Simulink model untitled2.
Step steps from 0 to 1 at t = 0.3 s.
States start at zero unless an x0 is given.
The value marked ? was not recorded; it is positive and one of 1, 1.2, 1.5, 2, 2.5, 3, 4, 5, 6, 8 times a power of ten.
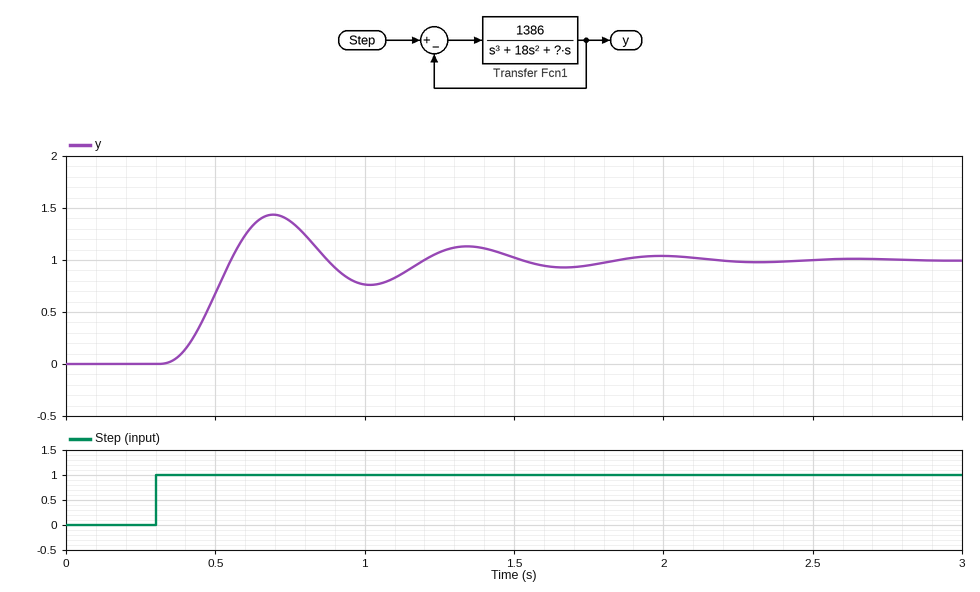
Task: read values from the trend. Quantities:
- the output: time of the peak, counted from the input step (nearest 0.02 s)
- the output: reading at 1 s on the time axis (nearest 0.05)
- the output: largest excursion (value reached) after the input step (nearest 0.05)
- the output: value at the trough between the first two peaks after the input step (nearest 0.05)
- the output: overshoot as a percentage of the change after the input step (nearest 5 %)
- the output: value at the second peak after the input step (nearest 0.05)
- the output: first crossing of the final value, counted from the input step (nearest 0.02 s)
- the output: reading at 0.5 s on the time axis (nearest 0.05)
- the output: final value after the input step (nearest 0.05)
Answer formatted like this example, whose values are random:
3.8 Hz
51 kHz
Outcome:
0.40 s
0.75
1.45
0.75
45 %
1.15
0.26 s
0.70
1.00
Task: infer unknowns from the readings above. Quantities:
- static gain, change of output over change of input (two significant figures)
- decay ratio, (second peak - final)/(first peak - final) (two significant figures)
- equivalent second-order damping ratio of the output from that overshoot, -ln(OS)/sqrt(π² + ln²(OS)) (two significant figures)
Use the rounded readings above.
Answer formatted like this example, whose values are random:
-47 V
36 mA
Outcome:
1.0
0.33
0.25
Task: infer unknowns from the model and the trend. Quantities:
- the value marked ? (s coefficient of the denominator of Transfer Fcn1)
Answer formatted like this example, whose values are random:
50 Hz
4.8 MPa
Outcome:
150
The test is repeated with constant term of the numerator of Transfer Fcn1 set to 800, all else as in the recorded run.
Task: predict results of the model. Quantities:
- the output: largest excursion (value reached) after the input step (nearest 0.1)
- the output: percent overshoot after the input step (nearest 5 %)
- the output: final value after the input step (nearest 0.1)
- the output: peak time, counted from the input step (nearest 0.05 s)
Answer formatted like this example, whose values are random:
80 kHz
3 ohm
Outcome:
1.2
15 %
1.0
0.50 s
